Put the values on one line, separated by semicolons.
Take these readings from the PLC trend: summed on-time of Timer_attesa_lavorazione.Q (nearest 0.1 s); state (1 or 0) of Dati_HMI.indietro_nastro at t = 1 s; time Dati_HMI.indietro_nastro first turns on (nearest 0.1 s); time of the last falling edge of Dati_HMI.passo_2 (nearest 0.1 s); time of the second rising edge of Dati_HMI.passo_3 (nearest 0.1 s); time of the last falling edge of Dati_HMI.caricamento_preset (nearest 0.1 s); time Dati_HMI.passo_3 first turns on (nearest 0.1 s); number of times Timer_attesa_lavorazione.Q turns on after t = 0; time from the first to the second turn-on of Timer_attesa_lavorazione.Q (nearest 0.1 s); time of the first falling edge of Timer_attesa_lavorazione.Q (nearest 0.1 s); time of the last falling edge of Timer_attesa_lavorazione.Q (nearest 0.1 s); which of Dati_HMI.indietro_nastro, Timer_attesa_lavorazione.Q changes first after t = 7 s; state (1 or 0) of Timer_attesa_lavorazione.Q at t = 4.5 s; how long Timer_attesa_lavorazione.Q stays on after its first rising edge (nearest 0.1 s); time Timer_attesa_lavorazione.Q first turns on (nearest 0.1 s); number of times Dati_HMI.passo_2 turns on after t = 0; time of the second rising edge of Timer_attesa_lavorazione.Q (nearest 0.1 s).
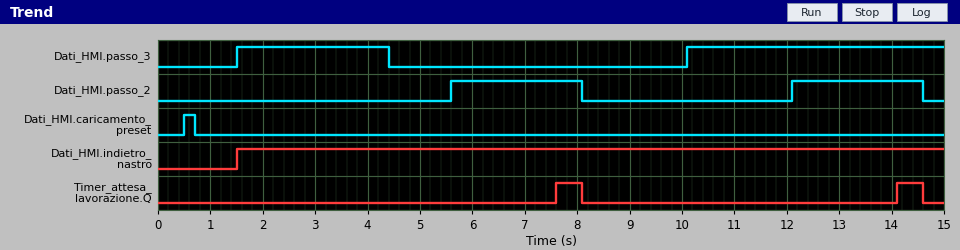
1.0 s; 0; 1.5 s; 14.6 s; 10.1 s; 0.7 s; 1.5 s; 2; 6.5 s; 8.1 s; 14.6 s; Timer_attesa_lavorazione.Q; 0; 0.5 s; 7.6 s; 2; 14.1 s
